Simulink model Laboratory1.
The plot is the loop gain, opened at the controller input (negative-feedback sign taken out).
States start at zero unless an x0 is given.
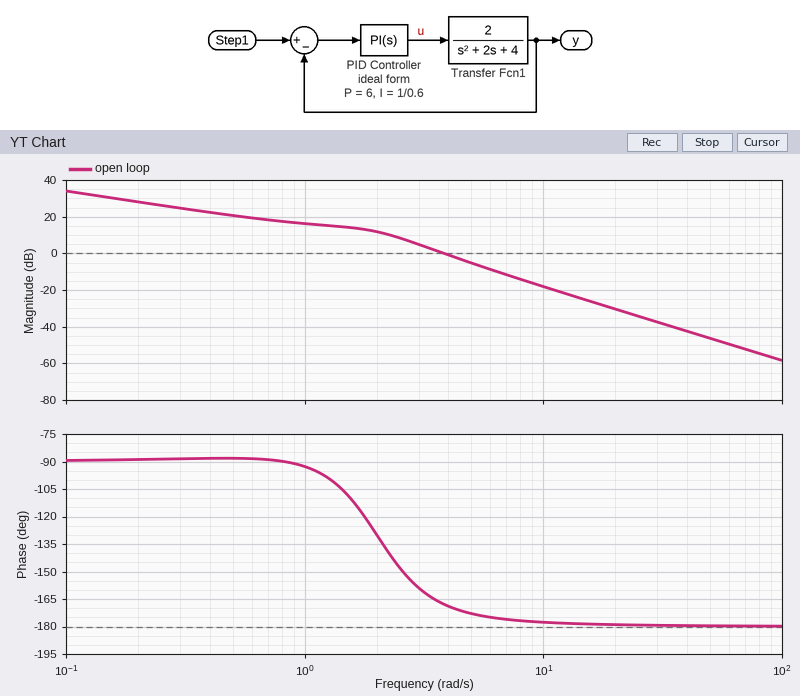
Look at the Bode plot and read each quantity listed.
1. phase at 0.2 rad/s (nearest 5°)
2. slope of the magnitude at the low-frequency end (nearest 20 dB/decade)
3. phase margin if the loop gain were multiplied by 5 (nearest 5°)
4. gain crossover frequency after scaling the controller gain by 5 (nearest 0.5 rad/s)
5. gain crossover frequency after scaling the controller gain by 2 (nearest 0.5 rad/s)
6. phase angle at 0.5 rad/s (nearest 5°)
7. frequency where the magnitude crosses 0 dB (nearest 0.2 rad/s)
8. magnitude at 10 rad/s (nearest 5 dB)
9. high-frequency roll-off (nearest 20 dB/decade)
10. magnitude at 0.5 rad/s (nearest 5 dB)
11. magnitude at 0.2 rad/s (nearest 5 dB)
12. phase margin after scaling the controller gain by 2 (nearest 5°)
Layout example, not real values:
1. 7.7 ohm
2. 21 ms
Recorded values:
1. -90°
2. -20 dB/decade
3. 5°
4. 8.0 rad/s
5. 5.0 rad/s
6. -90°
7. 3.8 rad/s
8. -20 dB
9. -40 dB/decade
10. 20 dB
11. 30 dB
12. 5°
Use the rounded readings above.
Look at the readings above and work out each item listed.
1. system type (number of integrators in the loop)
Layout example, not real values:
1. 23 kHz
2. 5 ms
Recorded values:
1. 1
